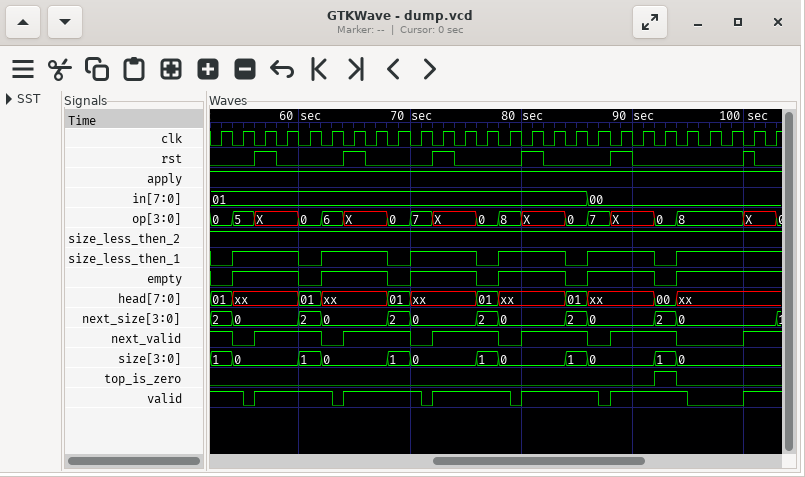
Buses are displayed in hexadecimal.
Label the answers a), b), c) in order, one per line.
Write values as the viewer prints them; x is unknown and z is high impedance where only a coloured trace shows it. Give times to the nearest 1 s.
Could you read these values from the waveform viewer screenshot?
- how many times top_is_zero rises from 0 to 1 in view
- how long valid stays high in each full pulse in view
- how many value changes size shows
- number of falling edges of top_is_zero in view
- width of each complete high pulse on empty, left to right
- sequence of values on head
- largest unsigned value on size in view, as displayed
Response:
a) 1
b) 7 s, 7 s, 7 s, 7 s, 7 s
c) 11
d) 1
e) 6 s, 6 s, 6 s, 6 s, 6 s
f) 01, xx, 01, xx, 01, xx, 01, xx, 01, xx, 00, xx
g) 1
